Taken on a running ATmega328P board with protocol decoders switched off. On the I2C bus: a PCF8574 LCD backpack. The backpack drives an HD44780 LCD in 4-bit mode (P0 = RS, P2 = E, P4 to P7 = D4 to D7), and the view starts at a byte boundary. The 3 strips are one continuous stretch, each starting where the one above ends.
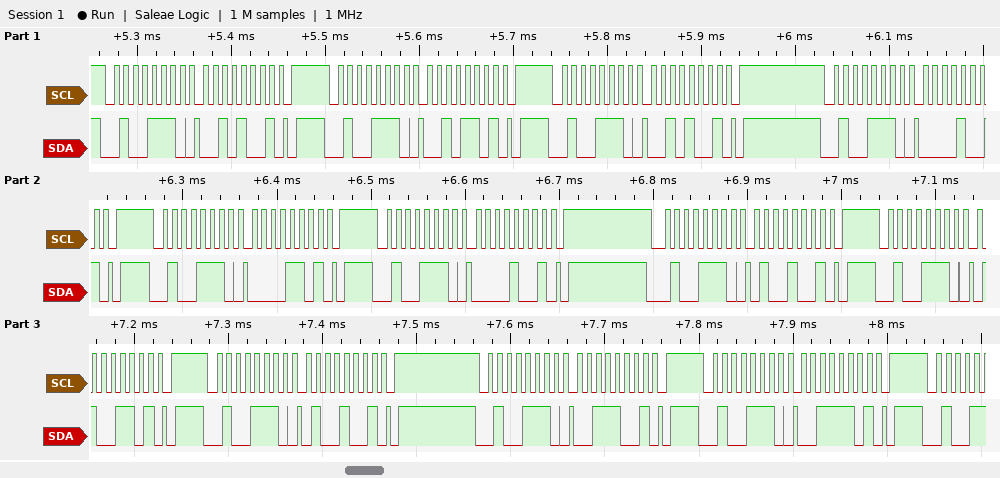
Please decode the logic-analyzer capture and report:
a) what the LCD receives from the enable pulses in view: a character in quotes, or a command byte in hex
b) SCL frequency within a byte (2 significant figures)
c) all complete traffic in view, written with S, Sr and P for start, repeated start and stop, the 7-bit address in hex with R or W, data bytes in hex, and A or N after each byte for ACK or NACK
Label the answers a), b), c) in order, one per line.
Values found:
a) ' '
b) 100 kHz
c) S 27W A 29 A P S 27W A 2D A P S 27W A 29 A P S 27W A 09 A P S 27W A 0D A P S 27W A 09 A P S 27W A 49 A P S 27W A 4D A P S 27W A 49 A P S 27W A 39 A P S 27W A 3D A P
